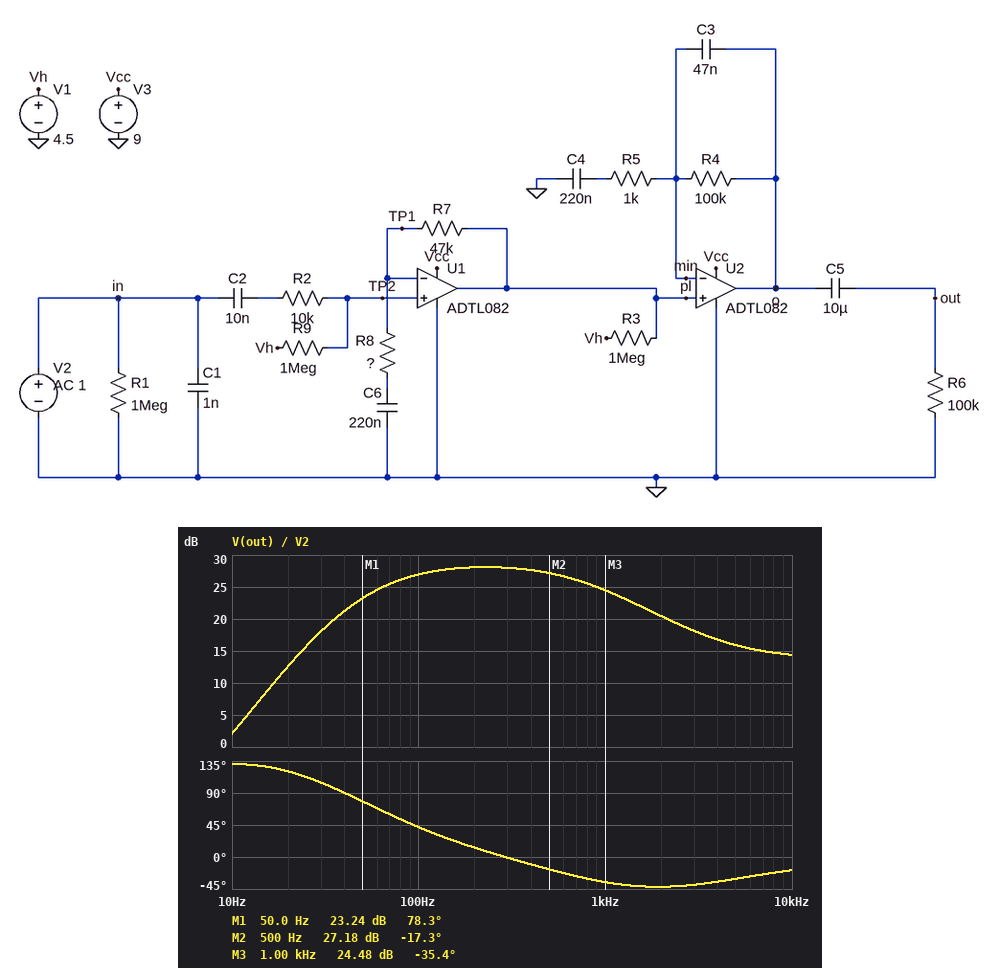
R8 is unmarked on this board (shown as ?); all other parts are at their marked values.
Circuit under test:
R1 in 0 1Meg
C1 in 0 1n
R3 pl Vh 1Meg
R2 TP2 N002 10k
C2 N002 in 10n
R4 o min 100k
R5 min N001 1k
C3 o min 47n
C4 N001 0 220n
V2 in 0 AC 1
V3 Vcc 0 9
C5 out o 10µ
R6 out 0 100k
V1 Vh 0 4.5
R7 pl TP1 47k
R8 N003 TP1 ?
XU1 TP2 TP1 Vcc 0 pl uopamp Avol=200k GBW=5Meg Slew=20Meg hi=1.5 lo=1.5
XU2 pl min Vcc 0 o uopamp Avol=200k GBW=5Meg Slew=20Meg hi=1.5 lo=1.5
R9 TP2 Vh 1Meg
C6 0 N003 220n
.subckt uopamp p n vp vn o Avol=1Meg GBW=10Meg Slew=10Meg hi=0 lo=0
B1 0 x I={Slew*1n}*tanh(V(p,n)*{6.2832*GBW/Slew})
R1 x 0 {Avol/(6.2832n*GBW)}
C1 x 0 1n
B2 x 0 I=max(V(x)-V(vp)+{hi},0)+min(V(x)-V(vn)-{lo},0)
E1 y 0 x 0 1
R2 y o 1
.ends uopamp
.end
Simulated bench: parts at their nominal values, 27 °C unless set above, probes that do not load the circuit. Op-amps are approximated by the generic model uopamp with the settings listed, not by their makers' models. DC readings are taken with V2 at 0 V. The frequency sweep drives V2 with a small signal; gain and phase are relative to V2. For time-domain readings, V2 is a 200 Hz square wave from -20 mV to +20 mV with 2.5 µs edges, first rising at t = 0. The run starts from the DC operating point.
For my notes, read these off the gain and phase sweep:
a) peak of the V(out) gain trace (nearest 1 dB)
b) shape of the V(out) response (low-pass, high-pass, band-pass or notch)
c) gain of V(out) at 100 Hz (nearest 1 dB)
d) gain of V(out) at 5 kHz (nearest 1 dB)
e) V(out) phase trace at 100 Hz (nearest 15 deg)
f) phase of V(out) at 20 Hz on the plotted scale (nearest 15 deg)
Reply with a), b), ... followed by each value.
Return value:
a) 28 dB
b) band-pass
c) 27 dB
d) 16 dB
e) 45 deg
f) 120 deg
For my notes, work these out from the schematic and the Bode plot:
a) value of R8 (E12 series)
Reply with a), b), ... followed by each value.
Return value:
a) 12 kΩ
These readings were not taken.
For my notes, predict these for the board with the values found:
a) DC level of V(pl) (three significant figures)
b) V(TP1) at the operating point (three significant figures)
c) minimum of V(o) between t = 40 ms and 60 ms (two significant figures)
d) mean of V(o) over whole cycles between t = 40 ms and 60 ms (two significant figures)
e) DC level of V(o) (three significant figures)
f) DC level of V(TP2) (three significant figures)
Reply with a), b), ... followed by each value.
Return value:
a) 4.50 V
b) 4.50 V
c) 3.8 V
d) 4.5 V
e) 4.50 V
f) 4.50 V
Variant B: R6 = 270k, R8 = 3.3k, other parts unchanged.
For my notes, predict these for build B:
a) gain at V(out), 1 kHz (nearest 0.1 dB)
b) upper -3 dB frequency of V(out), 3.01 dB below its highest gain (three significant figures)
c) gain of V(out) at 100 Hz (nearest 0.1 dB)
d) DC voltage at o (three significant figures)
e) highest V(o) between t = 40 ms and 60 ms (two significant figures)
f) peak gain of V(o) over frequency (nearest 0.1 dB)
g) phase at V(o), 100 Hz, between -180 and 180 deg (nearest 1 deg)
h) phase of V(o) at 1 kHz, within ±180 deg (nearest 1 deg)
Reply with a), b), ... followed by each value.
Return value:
a) 34.1 dB
b) 1.15 kHz
c) 30.5 dB
d) 4.50 V
e) 6.6 V
f) 36.4 dB
g) 75 deg
h) -27 deg
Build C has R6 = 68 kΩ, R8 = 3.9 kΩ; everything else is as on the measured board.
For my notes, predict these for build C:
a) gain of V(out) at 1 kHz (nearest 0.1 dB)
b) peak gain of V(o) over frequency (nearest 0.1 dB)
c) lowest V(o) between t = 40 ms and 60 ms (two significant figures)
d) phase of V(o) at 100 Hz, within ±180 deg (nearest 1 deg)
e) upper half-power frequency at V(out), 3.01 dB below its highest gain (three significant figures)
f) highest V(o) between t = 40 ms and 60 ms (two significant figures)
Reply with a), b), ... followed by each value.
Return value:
a) 32.8 dB
b) 35.4 dB
c) 2.7 V
d) 71 deg
e) 1.09 kHz
f) 6.3 V
